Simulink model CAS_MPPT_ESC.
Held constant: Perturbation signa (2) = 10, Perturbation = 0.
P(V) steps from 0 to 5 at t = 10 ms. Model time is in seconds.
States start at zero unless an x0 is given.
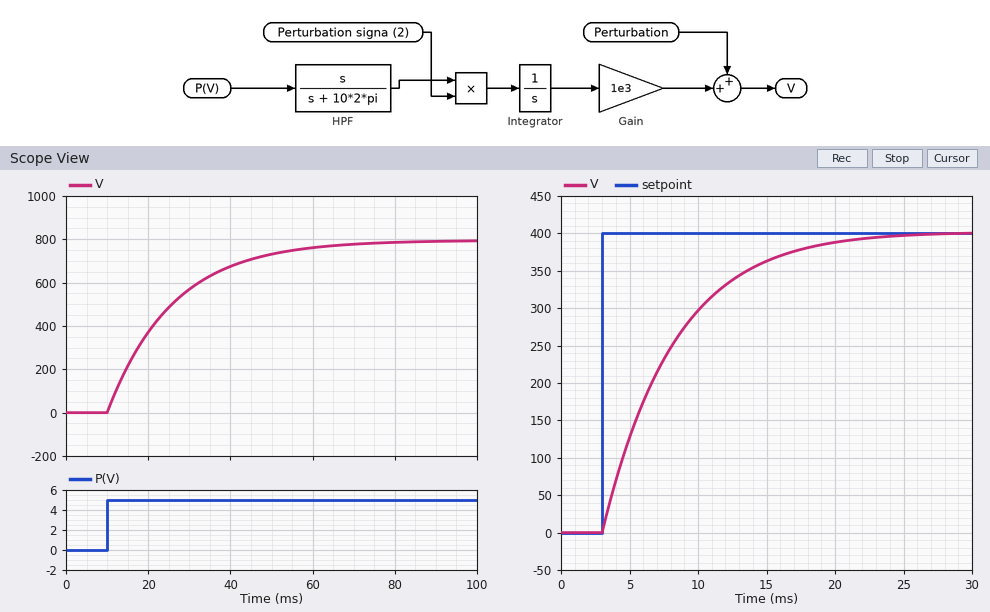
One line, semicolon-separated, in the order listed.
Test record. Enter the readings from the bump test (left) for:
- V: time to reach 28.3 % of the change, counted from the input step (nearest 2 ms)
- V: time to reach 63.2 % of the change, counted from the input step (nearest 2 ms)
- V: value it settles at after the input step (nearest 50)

6 ms; 16 ms; 800
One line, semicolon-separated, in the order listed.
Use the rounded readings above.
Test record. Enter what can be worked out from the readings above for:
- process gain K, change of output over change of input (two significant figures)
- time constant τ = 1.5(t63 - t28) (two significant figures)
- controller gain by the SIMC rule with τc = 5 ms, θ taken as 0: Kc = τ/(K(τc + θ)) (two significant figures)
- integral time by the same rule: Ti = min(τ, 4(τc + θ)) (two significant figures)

160; 15 ms; 0.019; 15 ms
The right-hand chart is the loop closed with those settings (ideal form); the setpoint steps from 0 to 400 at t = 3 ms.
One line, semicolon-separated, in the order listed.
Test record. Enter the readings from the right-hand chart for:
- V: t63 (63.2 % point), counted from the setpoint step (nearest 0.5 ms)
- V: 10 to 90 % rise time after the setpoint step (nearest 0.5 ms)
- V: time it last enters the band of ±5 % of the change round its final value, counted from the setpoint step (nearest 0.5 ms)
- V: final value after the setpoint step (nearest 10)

5.0 ms; 11.0 ms; 15.0 ms; 400
